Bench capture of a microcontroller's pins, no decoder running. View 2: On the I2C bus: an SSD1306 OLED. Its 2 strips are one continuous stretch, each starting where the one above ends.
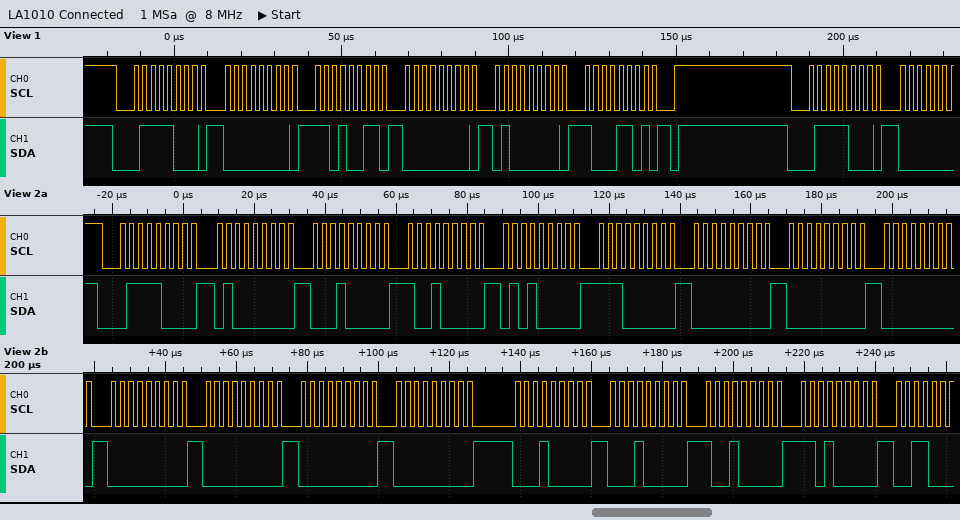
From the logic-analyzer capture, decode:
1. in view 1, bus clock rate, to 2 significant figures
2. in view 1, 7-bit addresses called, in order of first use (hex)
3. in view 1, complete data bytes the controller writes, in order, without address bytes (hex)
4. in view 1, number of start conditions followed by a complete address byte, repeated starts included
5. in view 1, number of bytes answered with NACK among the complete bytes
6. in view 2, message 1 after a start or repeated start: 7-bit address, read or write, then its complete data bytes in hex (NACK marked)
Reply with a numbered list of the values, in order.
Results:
1. 400 kHz
2. 0x3C
3. 00 D3 00 40 8D
4. 2
5. 0
6. 0x3C write: 40 10 90 50 E0 00 00 00 00 00 00 00 10 10 90 D0
